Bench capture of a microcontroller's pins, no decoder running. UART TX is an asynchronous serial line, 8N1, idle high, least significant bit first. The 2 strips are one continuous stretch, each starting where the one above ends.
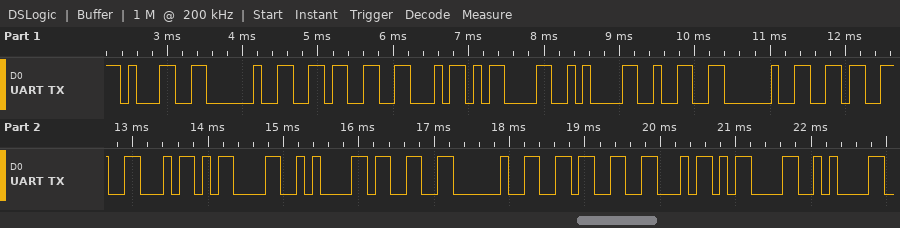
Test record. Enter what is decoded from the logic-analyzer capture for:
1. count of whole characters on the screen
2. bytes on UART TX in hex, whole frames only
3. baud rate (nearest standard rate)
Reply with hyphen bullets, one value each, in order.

- 18
- 0x31 0x20 0x36 0x46 0x0D 0x0A 0x32 0x20 0x36 0x46 0x0D 0x0A 0x33 0x20 0x36 0x46 0x0D 0x0A
- 9600 baud
